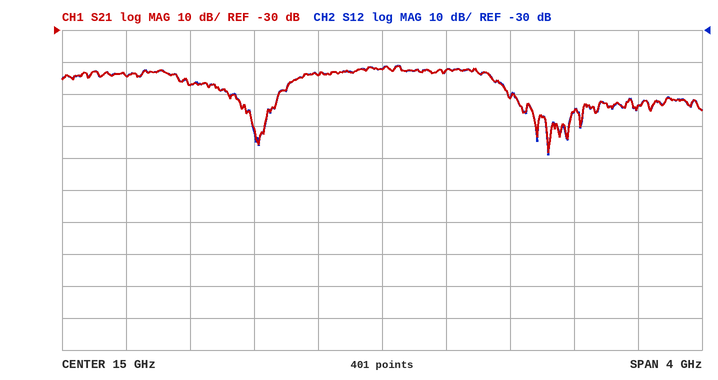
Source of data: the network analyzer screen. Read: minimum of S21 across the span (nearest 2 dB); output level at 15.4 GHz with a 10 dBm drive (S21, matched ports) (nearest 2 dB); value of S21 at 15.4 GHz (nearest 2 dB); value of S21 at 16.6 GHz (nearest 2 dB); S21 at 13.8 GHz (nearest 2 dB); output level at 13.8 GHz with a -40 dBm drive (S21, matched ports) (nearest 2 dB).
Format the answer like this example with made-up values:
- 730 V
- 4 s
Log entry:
- -68 dB
- -32 dBm
- -42 dB
- -54 dB
- -48 dB
- -88 dBm
